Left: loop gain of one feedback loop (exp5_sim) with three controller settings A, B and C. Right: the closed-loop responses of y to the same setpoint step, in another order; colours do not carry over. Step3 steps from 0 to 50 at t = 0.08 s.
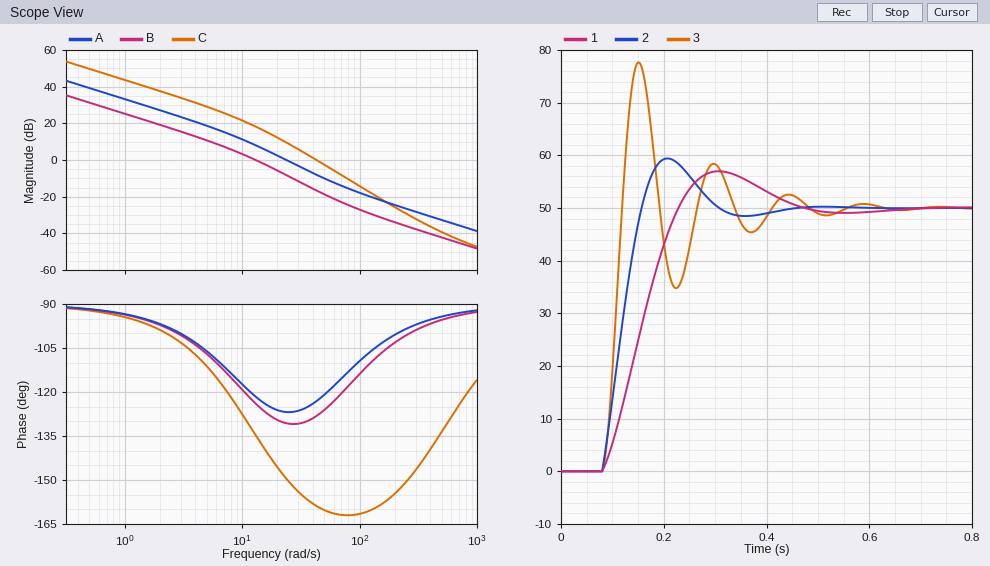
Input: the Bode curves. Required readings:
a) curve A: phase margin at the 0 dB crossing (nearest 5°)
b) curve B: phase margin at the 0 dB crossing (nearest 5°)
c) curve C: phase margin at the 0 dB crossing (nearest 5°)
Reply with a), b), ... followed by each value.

a) 55°
b) 55°
c) 20°
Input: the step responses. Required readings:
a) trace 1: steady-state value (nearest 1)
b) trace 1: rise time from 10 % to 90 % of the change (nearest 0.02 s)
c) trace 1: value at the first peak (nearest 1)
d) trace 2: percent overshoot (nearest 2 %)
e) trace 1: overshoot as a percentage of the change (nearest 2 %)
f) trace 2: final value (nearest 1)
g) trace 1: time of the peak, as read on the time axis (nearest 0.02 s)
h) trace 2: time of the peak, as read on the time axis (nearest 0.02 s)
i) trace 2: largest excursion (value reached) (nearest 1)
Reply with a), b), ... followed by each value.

a) 50
b) 0.10 s
c) 57
d) 18 %
e) 14 %
f) 50
g) 0.30 s
h) 0.20 s
i) 59
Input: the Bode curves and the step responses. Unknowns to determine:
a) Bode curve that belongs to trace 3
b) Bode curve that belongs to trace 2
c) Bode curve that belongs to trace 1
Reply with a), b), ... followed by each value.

a) C
b) A
c) B
